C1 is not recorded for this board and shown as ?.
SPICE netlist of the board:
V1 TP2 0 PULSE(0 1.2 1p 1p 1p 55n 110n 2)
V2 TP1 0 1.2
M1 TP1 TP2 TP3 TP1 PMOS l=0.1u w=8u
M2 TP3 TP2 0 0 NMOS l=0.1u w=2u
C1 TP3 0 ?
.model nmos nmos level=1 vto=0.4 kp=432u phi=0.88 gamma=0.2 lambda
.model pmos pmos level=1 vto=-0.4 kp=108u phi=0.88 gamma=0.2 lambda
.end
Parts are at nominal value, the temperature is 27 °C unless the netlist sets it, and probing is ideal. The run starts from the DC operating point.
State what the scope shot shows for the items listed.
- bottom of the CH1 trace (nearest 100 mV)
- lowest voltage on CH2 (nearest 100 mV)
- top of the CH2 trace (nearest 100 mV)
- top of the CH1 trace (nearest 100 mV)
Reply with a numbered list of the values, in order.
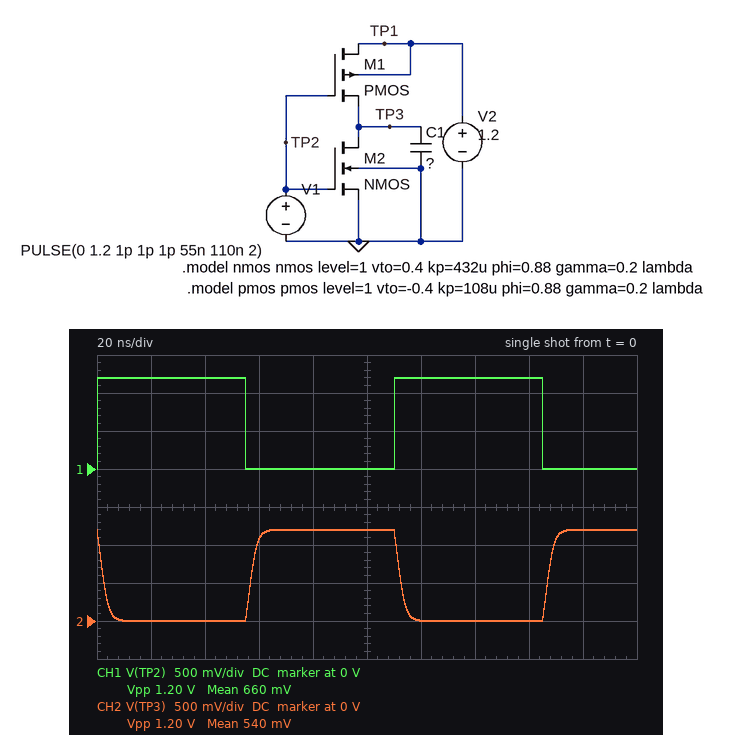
1. 0 V
2. 0 V
3. 1.2 V
4. 1.2 V
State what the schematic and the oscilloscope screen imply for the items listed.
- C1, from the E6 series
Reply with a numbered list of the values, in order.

1. 10 pF
